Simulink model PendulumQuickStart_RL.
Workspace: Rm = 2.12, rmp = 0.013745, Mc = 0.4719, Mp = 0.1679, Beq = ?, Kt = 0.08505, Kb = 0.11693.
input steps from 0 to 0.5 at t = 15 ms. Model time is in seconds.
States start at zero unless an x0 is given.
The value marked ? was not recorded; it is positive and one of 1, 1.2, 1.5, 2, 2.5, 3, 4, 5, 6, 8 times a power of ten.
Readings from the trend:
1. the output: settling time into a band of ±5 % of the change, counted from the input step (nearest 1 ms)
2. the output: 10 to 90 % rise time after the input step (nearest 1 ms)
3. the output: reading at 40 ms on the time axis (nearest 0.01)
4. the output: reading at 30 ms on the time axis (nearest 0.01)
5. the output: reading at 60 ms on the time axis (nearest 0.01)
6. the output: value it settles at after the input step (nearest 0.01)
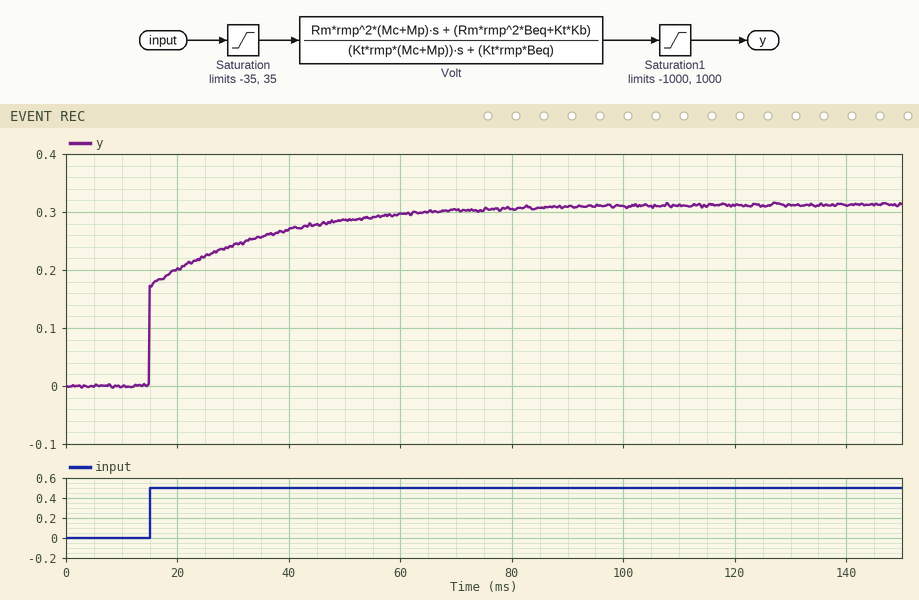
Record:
47 ms
32 ms
0.27
0.24
0.30
0.31
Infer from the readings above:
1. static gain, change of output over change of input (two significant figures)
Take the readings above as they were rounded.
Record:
0.62
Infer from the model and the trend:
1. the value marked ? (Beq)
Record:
30
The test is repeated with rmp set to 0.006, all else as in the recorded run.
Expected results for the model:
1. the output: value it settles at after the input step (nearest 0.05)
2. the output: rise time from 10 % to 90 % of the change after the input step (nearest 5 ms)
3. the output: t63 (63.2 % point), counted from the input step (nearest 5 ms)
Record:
0.40
45 ms
15 ms
